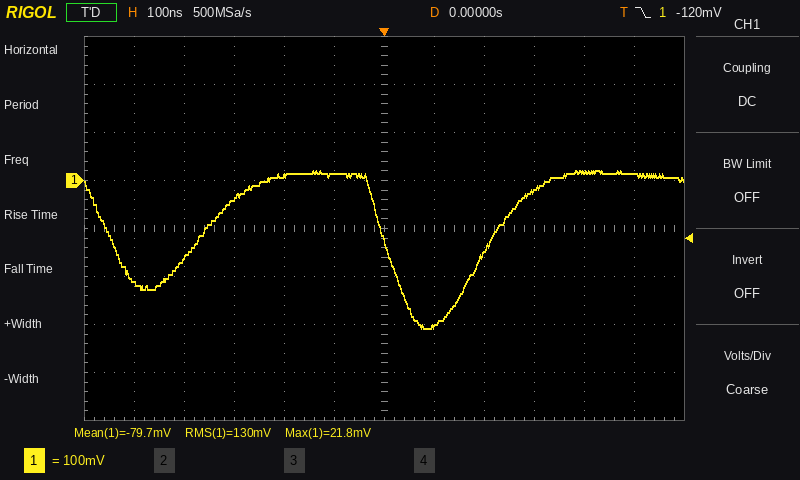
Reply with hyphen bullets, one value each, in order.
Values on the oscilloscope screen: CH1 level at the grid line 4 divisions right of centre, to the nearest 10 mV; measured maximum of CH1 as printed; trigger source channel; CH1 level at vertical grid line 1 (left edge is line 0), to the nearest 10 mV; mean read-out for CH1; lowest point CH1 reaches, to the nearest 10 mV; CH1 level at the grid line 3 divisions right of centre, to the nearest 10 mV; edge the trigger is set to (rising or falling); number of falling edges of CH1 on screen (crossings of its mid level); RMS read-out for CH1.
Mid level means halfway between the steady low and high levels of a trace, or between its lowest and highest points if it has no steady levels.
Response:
- 20 mV
- 21.8 mV
- CH1
- -210 mV
- -79.7 mV
- -310 mV
- -20 mV
- falling
- 2
- 130 mV
